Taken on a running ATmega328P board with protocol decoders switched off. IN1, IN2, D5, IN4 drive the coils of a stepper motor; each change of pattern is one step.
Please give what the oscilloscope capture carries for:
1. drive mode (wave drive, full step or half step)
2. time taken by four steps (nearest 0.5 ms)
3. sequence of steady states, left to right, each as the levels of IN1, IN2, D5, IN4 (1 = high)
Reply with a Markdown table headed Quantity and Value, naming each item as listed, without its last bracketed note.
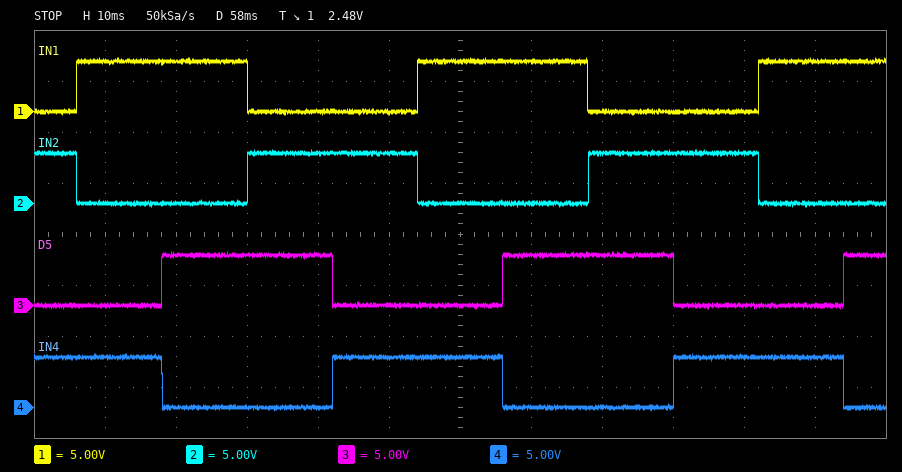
| Quantity | Value |
|---|---|
| drive mode | full step |
| time taken by four steps | 48.0 ms |
| sequence of steady states, left to right, each as the levels of IN1, IN2, D5, IN4 | 0101 1001 1010 0110 0101 1001 1010 0110 0101 1001 1010 |
